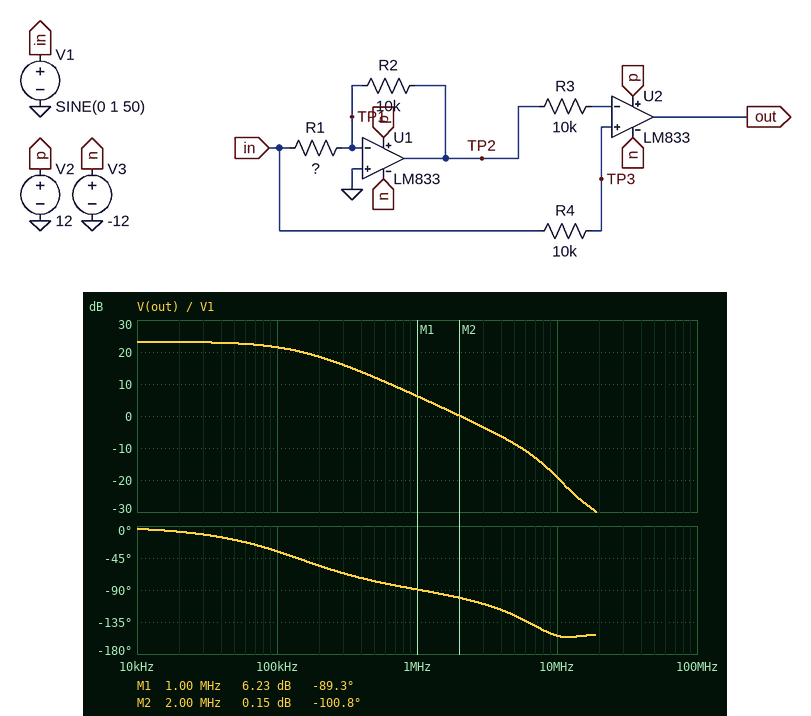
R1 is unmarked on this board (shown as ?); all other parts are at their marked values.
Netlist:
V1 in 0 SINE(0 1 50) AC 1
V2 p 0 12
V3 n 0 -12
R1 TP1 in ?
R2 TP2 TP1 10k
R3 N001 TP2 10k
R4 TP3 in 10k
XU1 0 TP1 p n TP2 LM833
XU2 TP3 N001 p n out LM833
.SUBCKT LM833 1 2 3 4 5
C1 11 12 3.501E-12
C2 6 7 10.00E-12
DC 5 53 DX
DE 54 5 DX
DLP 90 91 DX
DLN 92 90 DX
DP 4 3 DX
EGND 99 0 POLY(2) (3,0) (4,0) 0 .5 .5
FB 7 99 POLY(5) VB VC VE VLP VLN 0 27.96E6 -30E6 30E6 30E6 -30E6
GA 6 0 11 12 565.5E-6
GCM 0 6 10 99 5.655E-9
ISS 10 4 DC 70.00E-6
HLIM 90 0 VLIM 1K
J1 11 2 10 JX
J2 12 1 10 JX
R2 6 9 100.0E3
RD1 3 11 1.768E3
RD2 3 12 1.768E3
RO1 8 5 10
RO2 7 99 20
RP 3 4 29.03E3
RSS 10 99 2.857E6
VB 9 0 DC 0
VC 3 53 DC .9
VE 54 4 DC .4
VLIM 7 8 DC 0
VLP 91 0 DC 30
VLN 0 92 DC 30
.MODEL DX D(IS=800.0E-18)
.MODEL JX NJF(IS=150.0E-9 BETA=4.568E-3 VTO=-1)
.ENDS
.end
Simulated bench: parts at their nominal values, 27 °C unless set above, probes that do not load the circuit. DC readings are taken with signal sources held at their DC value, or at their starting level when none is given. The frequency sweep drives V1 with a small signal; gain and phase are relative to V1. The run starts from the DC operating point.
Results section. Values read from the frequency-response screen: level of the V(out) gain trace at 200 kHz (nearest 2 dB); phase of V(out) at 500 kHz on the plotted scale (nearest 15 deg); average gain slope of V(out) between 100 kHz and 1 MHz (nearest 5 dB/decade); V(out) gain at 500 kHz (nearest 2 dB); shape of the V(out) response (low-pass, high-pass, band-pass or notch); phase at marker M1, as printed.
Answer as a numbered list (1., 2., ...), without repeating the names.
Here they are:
1. 18 dB
2. -75 deg
3. -15 dB/decade
4. 12 dB
5. low-pass
6. -89.3 deg
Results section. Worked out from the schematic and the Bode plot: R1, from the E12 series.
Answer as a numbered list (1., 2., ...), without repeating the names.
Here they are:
1. 15 kΩ
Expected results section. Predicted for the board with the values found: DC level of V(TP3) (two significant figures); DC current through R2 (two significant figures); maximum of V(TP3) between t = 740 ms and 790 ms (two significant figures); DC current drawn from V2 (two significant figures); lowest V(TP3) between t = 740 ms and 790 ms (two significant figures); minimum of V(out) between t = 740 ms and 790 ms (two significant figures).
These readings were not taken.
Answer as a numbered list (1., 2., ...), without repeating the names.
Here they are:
1. 3.0 mV
2. 300 nA
3. 1.0 V
4. 1.8 mA
5. -1.0 V
6. -12 V
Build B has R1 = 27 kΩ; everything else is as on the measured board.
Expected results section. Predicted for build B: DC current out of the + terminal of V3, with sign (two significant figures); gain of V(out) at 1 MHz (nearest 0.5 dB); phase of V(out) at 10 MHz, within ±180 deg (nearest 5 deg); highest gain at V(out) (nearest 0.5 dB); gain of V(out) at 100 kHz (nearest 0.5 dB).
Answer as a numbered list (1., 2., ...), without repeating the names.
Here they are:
1. -1.8 mA
2. 4.5 dB
3. -145 deg
4. 21.5 dB
5. 20.0 dB
